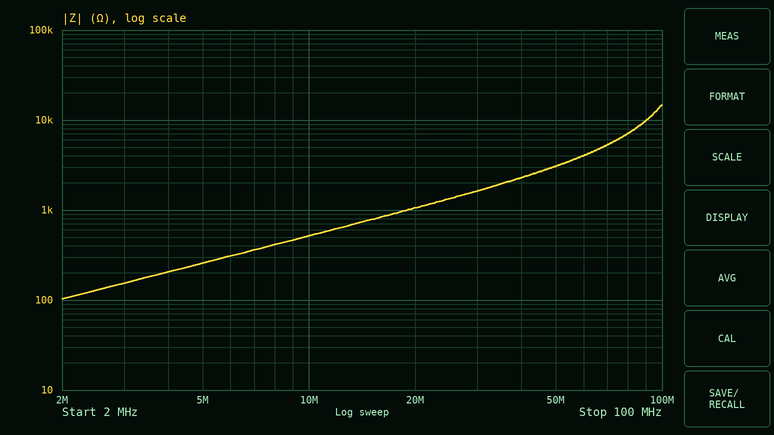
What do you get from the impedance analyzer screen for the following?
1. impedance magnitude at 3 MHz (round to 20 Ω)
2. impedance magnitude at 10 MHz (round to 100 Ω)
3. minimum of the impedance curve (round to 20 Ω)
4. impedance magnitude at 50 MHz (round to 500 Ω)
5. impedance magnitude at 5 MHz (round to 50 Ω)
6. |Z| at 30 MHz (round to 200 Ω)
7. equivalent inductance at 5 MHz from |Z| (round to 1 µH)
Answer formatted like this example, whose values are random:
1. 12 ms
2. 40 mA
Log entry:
1. 160 Ω
2. 500 Ω
3. 100 Ω
4. 3.0 kΩ
5. 250 Ω
6. 1.6 kΩ
7. 8 µH
